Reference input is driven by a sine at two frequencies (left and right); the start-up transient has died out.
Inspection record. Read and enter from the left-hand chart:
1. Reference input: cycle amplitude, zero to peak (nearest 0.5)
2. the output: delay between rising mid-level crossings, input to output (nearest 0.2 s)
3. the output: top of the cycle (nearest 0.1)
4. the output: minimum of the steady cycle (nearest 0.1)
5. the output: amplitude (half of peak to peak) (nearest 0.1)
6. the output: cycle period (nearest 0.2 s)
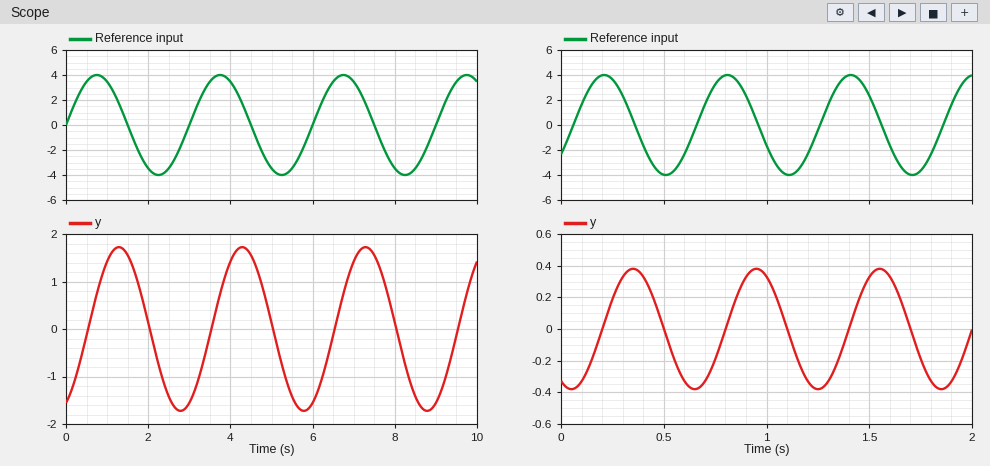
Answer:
4.0
0.6 s
1.7
-1.7
1.7
3.0 s
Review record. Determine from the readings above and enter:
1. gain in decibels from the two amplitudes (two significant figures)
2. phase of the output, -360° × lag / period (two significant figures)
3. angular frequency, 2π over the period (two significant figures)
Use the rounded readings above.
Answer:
-7.4 dB
-72°
2.1 rad/s
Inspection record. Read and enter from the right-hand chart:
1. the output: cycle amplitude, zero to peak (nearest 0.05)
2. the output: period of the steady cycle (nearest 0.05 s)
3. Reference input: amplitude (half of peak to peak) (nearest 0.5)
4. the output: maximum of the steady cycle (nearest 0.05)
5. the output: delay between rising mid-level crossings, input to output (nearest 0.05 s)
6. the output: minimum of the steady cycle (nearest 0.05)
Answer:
0.40
0.60 s
4.0
0.40
0.15 s
-0.40
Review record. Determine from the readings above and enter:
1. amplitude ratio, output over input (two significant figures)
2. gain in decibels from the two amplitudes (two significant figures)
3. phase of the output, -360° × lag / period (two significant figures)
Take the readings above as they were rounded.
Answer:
0.10
-20 dB
-90°
